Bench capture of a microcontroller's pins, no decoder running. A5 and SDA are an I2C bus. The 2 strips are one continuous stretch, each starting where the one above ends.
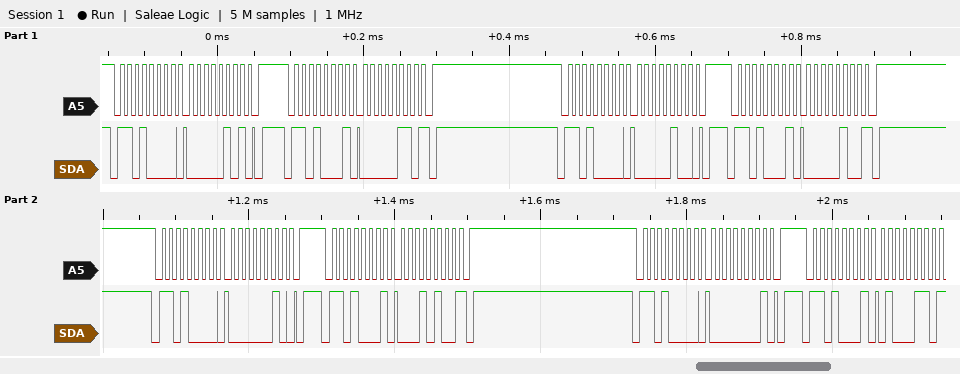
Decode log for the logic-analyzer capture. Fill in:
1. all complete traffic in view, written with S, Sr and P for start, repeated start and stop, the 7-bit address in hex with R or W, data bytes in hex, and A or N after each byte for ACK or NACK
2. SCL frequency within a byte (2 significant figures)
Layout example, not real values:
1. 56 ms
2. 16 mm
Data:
1. S 68W A 05 A P S 68R A 06 N P S 68W A 04 A P S 68R A 04 N P S 68W A 02 A P S 68R A 14 N P S 68W A 01 A P S 68R A 46 N
2. 100 kHz
